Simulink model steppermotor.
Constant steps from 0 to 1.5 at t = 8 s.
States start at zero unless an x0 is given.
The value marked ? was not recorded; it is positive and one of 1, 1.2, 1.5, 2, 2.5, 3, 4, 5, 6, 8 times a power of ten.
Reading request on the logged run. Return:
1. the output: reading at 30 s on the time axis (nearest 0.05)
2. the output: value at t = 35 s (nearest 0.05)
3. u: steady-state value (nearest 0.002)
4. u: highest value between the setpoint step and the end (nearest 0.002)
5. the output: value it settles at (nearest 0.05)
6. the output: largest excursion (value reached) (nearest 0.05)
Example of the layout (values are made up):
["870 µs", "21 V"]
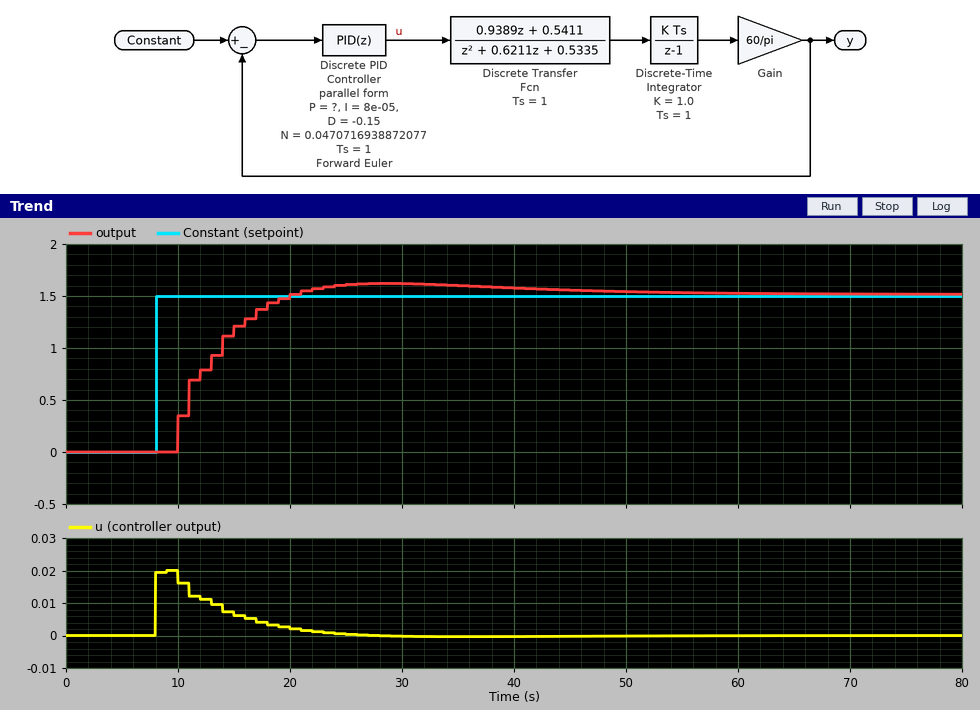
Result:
["1.60", "1.60", "0.000", "0.020", "1.50", "1.60"]
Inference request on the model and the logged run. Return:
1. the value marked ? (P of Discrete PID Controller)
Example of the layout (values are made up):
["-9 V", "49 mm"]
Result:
["0.02"]
